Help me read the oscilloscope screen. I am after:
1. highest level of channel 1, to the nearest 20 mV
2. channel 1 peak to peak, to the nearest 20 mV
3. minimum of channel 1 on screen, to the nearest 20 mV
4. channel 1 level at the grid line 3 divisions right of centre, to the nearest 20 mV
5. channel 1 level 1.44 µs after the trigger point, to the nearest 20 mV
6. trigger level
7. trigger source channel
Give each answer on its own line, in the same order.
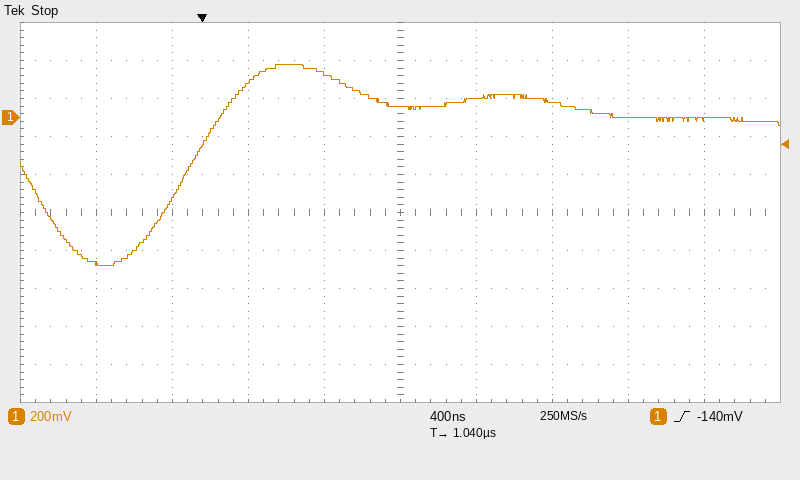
280 mV
1.06 V
-780 mV
0 mV
100 mV
-140 mV
channel 1
